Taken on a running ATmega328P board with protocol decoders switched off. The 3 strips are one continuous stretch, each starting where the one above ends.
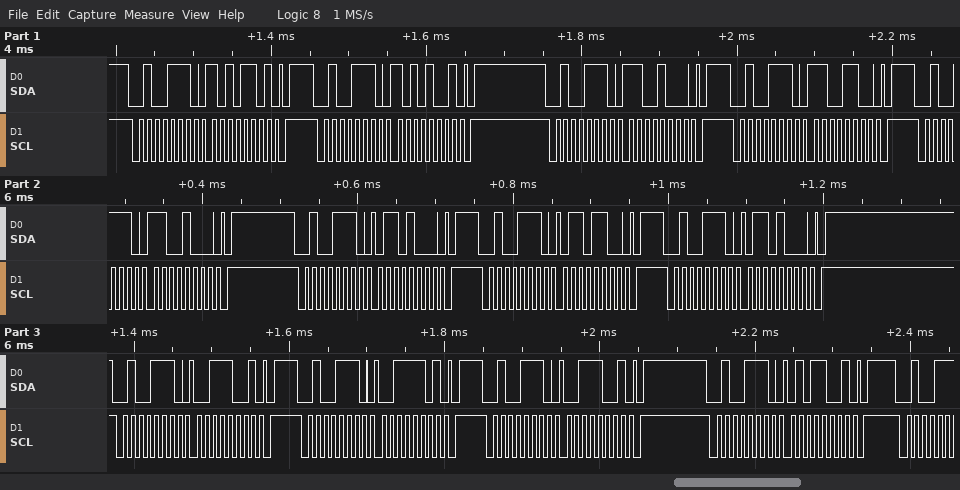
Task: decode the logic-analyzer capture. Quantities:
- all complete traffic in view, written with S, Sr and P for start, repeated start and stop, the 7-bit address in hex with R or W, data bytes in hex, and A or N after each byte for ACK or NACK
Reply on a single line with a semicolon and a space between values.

S 27W A AD A P S 27W A A9 A P S 27W A C8 A P S 27W A CC A P S 27W A C8 A P S 27W A 68 A P S 27W A 6C A P S 27W A 68 A P S 27W A 39 A P S 27W A 3D A P S 27W A 39 A P S 27W A 59 A P
